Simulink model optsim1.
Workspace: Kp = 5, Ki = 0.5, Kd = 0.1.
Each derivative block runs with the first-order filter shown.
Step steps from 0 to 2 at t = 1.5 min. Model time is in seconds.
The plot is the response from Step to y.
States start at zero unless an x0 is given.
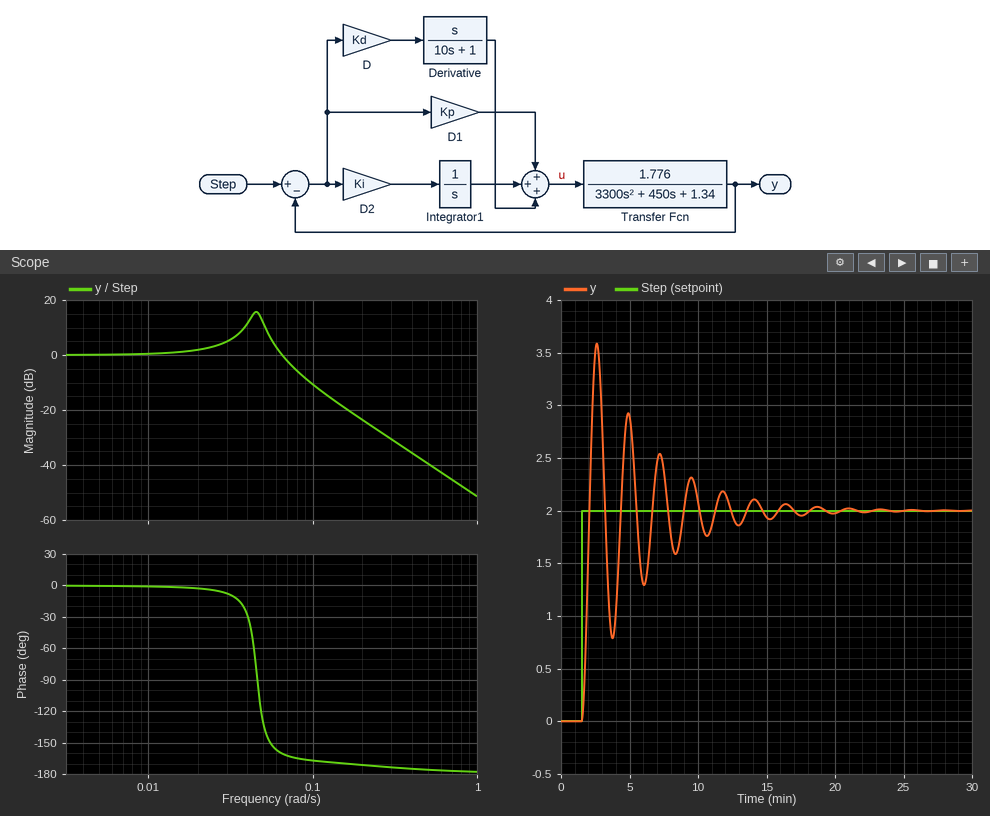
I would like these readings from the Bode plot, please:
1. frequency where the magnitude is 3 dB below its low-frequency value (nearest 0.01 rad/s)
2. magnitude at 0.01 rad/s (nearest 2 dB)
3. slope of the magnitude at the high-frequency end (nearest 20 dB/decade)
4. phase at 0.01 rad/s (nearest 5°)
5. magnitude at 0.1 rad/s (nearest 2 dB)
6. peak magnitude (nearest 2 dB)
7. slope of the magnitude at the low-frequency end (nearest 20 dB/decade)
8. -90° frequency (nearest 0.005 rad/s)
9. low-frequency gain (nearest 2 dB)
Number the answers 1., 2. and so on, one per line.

1. 0.07 rad/s
2. 0 dB
3. -40 dB/decade
4. 0°
5. -10 dB
6. 16 dB
7. 0 dB/decade
8. 0.045 rad/s
9. 0 dB
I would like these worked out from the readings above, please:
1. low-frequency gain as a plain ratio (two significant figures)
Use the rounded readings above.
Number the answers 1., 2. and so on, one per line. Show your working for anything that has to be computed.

1. 10^(0 / 20) = 1.0
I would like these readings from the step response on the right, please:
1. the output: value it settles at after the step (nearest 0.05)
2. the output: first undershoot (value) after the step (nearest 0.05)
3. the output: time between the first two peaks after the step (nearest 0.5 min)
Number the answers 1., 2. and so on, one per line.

1. 2.00
2. 0.80
3. 2.5 min
